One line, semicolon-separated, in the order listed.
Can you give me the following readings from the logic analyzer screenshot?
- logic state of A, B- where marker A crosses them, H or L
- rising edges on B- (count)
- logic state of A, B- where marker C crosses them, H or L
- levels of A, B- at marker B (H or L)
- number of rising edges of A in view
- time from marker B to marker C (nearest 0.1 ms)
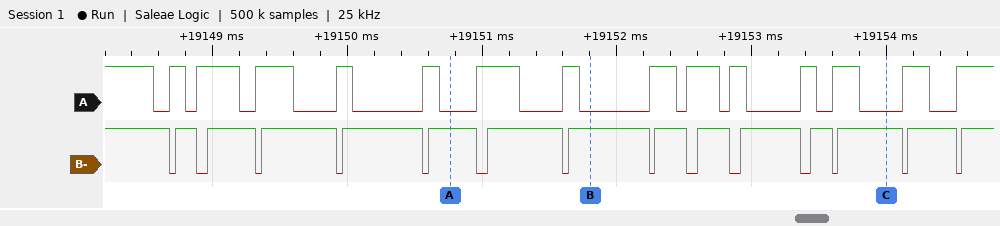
A=L, B-=H; 14; A=L, B-=H; A=L, B-=H; 14; 2.2 ms
